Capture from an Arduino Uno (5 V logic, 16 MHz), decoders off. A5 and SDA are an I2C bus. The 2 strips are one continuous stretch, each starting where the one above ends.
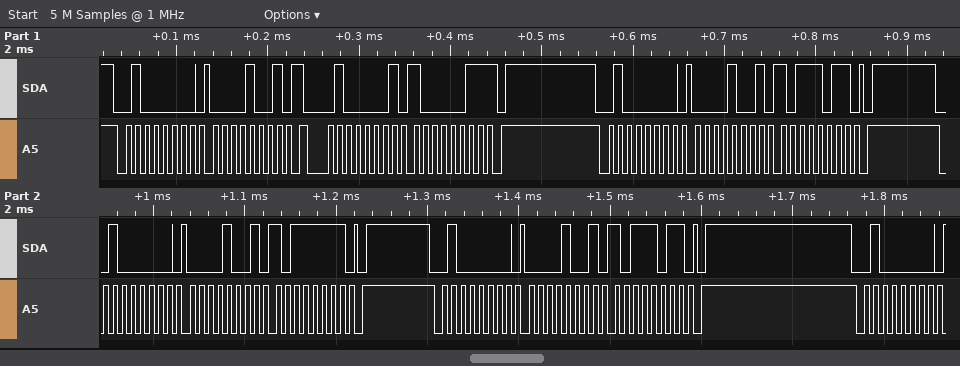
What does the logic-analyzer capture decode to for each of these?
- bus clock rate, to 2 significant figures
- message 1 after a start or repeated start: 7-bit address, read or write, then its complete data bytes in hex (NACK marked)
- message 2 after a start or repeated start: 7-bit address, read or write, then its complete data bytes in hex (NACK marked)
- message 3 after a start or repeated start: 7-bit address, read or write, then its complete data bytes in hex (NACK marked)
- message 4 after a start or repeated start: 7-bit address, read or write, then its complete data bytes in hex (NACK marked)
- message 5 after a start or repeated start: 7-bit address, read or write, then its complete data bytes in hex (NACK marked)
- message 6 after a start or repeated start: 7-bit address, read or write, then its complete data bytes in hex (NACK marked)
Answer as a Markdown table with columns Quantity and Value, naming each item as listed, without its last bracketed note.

| Quantity | Value |
|---|---|
| bus clock rate, to 2 significant figures | 100 kHz |
| message 1 after a start or repeated start: 7-bit address, read or write, then its complete data bytes in hex | 0x20 write: 09 |
| message 2 after a start or repeated start: 7-bit address, read or write, then its complete data bytes in hex | 0x20 read: 83 NACK |
| message 3 after a start or repeated start: 7-bit address, read or write, then its complete data bytes in hex | 0x20 write: 09 BB |
| message 4 after a start or repeated start: 7-bit address, read or write, then its complete data bytes in hex | 0x20 write: 09 BF |
| message 5 after a start or repeated start: 7-bit address, read or write, then its complete data bytes in hex | 0x20 write: 09 BB |
| message 6 after a start or repeated start: 7-bit address, read or write, then its complete data bytes in hex | 0x20 write |
